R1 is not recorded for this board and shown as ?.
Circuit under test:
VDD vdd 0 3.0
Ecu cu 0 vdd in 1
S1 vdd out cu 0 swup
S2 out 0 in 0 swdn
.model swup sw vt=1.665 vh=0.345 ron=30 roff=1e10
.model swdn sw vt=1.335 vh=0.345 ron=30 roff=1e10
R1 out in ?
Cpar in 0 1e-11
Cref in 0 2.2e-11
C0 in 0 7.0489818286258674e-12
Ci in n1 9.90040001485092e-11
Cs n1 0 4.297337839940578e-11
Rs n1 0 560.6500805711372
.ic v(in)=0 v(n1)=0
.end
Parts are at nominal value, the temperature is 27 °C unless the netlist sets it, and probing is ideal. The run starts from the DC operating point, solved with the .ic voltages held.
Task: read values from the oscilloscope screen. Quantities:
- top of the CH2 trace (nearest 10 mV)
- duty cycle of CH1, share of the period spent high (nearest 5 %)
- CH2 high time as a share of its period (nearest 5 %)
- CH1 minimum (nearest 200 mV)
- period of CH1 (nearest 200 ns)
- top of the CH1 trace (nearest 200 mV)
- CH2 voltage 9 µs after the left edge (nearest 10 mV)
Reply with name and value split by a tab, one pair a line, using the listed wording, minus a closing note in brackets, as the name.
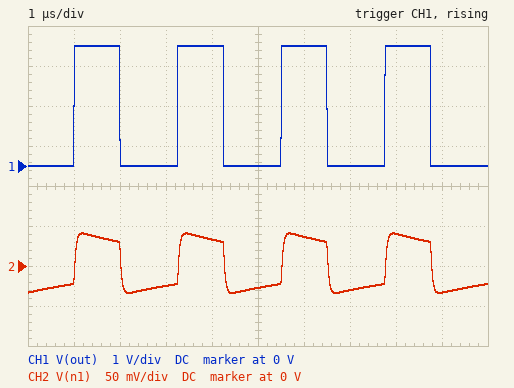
top of the CH2 trace	40 mV
duty cycle of CH1, share of the period spent high	45 %
CH2 high time as a share of its period	45 %
CH1 minimum	0 V
period of CH1	2.2 µs
top of the CH1 trace	3.0 V
CH2 voltage 9 µs after the left edge	-30 mV
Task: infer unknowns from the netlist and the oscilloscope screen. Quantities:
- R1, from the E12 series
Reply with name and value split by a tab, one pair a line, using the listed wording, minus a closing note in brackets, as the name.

R1, from the E12 series	18 kΩ
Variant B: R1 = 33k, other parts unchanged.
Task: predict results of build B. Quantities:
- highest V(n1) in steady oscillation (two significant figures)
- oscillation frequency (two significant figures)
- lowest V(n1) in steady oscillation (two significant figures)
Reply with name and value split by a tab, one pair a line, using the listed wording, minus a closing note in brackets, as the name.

highest V(n1) in steady oscillation	23 mV
oscillation frequency	240 kHz
lowest V(n1) in steady oscillation	-19 mV
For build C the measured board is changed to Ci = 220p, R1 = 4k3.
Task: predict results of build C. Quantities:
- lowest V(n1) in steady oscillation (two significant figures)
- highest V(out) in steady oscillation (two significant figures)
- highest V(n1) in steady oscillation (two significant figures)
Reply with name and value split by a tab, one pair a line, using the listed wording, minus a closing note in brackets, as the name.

lowest V(n1) in steady oscillation	-140 mV
highest V(out) in steady oscillation	3.0 V
highest V(n1) in steady oscillation	170 mV
